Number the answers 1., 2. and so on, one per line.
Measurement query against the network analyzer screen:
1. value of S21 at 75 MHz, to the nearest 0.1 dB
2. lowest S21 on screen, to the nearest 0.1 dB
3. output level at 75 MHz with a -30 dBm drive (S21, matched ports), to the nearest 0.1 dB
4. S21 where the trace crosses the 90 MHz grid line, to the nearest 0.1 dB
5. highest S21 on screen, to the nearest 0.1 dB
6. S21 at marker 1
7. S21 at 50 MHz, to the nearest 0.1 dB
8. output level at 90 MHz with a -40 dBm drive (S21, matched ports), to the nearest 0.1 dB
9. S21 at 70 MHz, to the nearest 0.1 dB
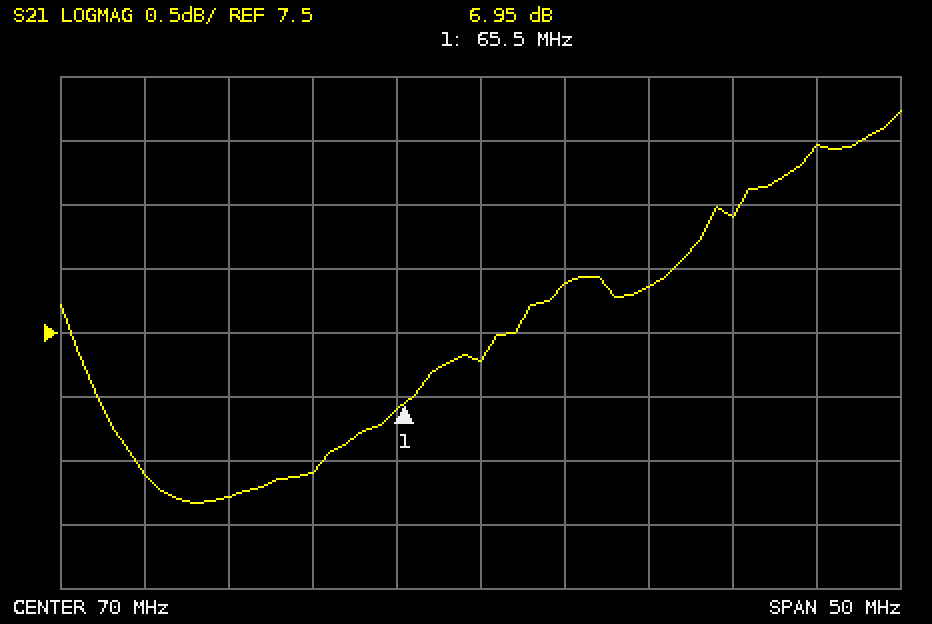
1. 7.9 dB
2. 6.2 dB
3. -22.1 dBm
4. 9.0 dB
5. 9.2 dB
6. 6.95 dB
7. 6.4 dB
8. -31.0 dBm
9. 7.3 dB
